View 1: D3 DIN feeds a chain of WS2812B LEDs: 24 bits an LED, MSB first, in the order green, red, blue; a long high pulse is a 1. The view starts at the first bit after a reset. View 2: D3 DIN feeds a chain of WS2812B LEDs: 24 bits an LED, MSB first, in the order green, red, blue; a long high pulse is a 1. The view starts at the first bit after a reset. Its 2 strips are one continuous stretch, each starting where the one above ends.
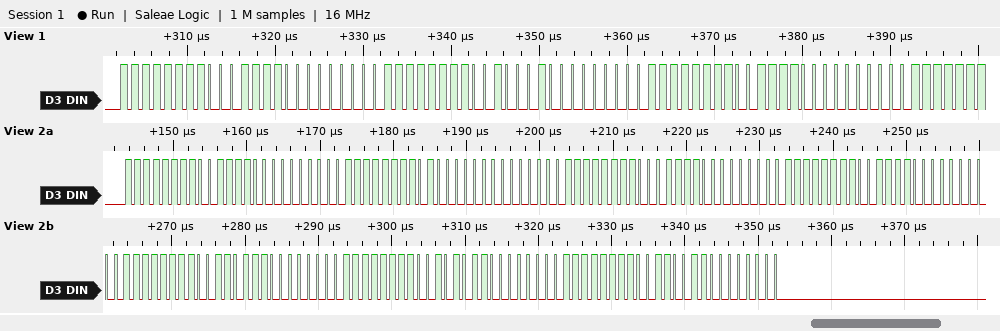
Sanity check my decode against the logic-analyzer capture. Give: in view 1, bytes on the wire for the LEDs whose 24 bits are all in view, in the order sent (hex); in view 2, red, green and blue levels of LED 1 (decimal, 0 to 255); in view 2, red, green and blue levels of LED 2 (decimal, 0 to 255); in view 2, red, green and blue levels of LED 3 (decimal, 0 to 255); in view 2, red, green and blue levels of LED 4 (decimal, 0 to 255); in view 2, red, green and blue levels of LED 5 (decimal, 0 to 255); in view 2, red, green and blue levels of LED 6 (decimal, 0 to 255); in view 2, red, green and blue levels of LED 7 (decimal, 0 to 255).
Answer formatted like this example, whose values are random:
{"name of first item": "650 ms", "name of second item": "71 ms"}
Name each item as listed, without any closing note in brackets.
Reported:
{"in view 1, bytes on the wire for the LEDs whose 24 bits are all in view, in the order sent": "FF 1E 00 FF 22 00 FF 3C 00", "in view 2, red, green and blue levels of LED 1": "60, 255, 0", "in view 2, red, green and blue levels of LED 2": "64, 255, 0", "in view 2, red, green and blue levels of LED 3": "30, 255, 0", "in view 2, red, green and blue levels of LED 4": "60, 255, 0", "in view 2, red, green and blue levels of LED 5": "55, 255, 0", "in view 2, red, green and blue levels of LED 6": "43, 255, 0", "in view 2, red, green and blue levels of LED 7": "51, 255, 0"}
